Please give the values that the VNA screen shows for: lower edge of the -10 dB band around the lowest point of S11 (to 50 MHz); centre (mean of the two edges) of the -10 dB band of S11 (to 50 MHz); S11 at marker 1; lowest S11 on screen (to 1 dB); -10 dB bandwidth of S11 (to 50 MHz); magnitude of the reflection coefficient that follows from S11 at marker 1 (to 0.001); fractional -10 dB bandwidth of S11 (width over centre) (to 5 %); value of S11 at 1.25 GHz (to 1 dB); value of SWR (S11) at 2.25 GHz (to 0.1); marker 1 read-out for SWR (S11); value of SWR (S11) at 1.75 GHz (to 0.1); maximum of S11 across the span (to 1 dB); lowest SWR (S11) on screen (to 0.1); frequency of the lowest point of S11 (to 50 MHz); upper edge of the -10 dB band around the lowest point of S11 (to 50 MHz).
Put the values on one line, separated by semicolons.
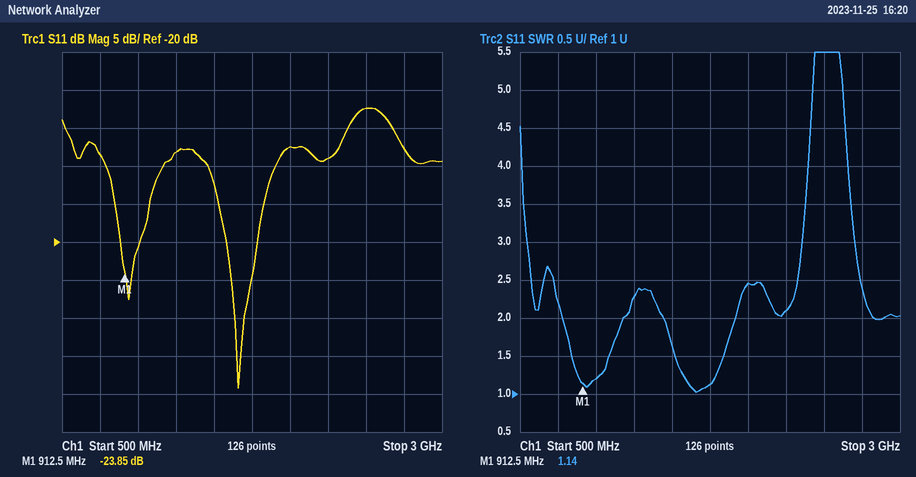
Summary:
1.45 GHz; 1.70 GHz; -23.85 dB; -39 dB; 450 MHz; 0.064; 25 %; -8 dB; 2.1; 1.14; 1.1; -2 dB; 1.0; 1.65 GHz; 1.90 GHz
